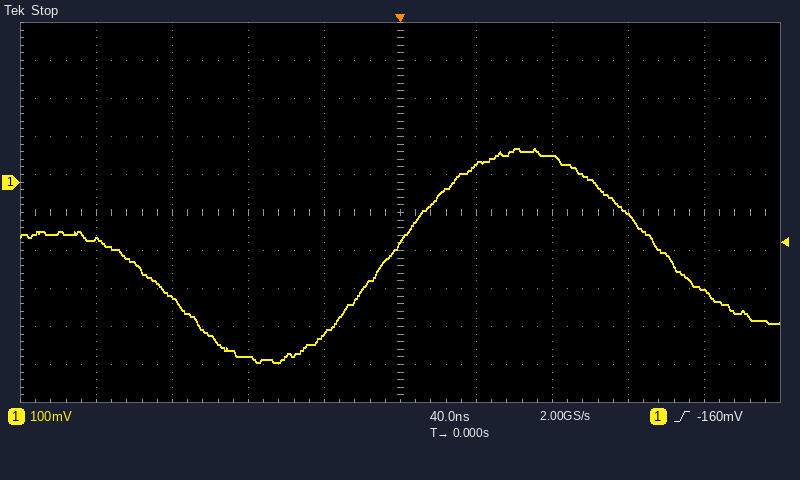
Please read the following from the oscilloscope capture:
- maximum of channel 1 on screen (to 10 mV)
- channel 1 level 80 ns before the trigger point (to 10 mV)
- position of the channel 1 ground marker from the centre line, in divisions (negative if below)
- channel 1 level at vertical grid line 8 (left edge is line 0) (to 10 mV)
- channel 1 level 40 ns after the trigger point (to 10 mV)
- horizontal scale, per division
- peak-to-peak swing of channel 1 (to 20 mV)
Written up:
90 mV
-460 mV
+0.8 div
-80 mV
50 mV
40 ns
560 mV
